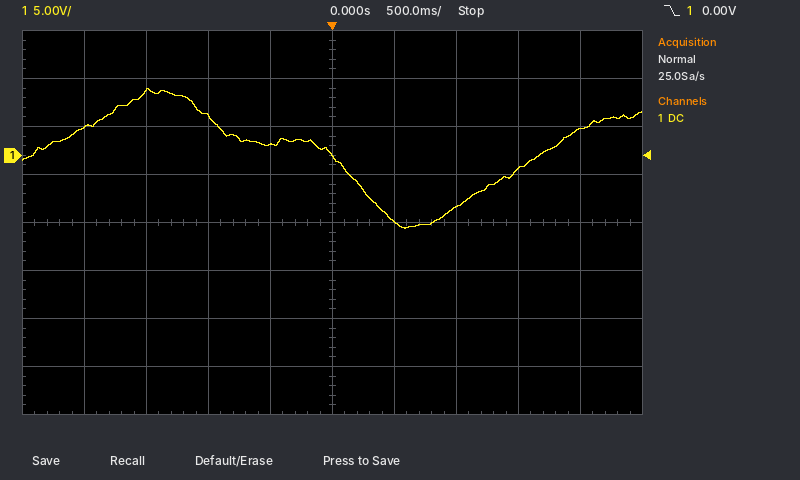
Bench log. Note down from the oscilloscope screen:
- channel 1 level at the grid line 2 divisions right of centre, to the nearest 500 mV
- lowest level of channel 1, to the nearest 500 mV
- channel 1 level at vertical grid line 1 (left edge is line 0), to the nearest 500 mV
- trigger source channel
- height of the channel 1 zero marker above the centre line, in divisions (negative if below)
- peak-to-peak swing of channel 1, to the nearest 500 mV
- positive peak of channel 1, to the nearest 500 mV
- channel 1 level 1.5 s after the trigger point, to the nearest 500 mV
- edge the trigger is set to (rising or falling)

-5.5 V
-7.5 V
3.0 V
channel 1
+1.4 div
14.5 V
7.0 V
-1.5 V
falling
